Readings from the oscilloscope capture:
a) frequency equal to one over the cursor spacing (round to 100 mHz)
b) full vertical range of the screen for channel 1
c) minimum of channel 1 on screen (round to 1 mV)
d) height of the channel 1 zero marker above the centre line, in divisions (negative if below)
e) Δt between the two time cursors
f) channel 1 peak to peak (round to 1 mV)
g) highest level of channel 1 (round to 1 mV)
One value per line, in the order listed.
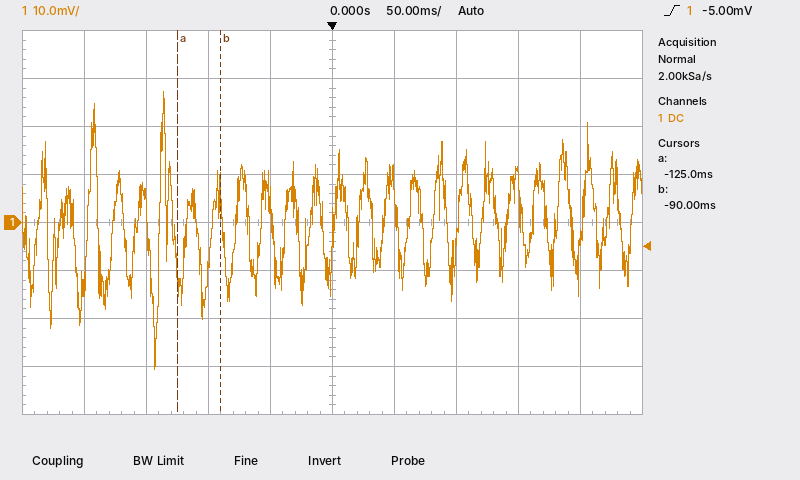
28.6 Hz
80 mV
-31 mV
0.0 div
35 ms
58 mV
27 mV
